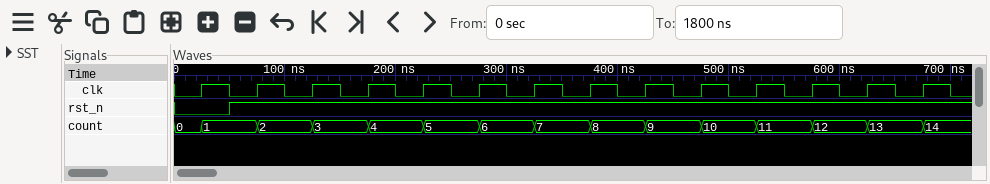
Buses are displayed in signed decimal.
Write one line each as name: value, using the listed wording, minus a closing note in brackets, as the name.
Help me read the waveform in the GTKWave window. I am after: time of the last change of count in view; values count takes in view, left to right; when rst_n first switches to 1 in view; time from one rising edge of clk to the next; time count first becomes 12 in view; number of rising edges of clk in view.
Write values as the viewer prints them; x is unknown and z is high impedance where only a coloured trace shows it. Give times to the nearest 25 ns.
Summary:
time of the last change of count in view: 675 ns
values count takes in view, left to right: 0, 1, 2, 3, 4, 5, 6, 7, 8, 9, 10, 11, 12, 13, 14
when rst_n first switches to 1 in view: 50 ns
time from one rising edge of clk to the next: 50 ns
time count first becomes 12 in view: 575 ns
number of rising edges of clk in view: 14
